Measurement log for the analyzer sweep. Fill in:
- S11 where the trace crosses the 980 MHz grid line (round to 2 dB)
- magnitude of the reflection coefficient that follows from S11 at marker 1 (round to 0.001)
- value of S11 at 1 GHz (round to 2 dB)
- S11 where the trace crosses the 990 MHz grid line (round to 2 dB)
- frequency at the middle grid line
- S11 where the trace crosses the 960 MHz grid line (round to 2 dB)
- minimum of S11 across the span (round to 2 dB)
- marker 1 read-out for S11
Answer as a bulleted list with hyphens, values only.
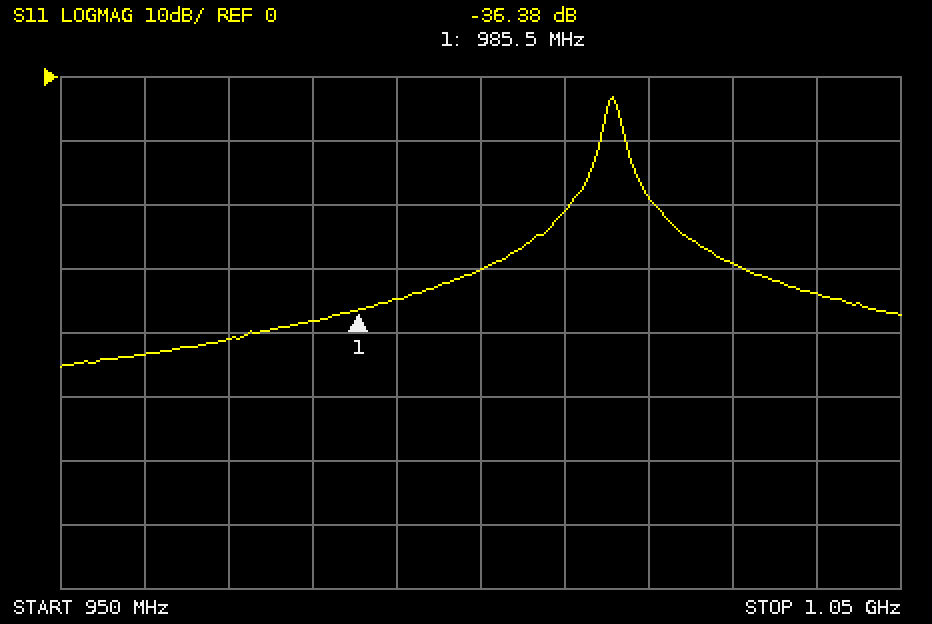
- -38 dB
- 0.015
- -30 dB
- -34 dB
- 1 GHz
- -44 dB
- -46 dB
- -36.38 dB
